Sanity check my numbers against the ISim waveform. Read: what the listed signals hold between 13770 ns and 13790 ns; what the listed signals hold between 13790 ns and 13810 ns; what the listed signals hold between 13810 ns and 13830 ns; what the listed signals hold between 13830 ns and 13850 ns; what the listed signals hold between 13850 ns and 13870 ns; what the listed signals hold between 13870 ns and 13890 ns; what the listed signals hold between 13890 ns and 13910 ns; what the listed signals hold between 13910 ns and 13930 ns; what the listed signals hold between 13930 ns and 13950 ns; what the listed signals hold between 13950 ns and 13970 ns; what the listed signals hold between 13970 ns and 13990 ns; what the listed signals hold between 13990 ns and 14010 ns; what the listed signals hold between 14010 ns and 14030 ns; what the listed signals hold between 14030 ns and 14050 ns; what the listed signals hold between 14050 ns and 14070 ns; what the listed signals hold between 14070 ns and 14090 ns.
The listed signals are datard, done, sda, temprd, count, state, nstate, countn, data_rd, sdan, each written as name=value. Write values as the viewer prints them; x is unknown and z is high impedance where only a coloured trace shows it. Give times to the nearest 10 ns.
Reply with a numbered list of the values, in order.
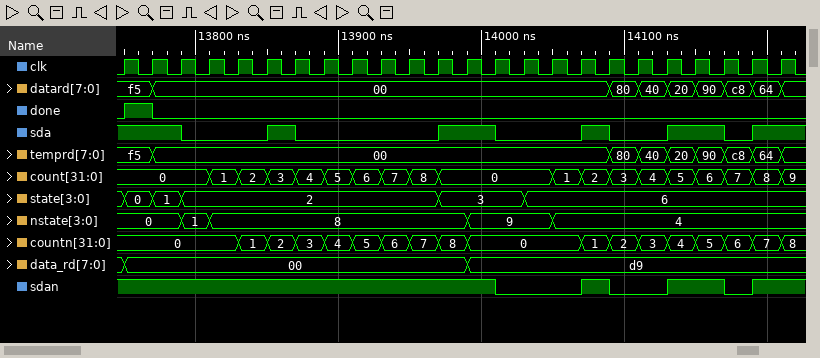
1. datard=00, done=0, sda=1, temprd=00, count=0, state=1, nstate=0, countn=0, data_rd=00, sdan=1
2. datard=00, done=0, sda=0, temprd=00, count=0, state=2, nstate=1, countn=0, data_rd=00, sdan=1
3. datard=00, done=0, sda=0, temprd=00, count=1, state=2, nstate=8, countn=0, data_rd=00, sdan=1
4. datard=00, done=0, sda=0, temprd=00, count=2, state=2, nstate=8, countn=1, data_rd=00, sdan=1
5. datard=00, done=0, sda=1, temprd=00, count=3, state=2, nstate=8, countn=2, data_rd=00, sdan=1
6. datard=00, done=0, sda=0, temprd=00, count=4, state=2, nstate=8, countn=3, data_rd=00, sdan=1
7. datard=00, done=0, sda=0, temprd=00, count=5, state=2, nstate=8, countn=4, data_rd=00, sdan=1
8. datard=00, done=0, sda=0, temprd=00, count=6, state=2, nstate=8, countn=5, data_rd=00, sdan=1
9. datard=00, done=0, sda=0, temprd=00, count=7, state=2, nstate=8, countn=6, data_rd=00, sdan=1
10. datard=00, done=0, sda=0, temprd=00, count=8, state=2, nstate=8, countn=7, data_rd=00, sdan=1
11. datard=00, done=0, sda=1, temprd=00, count=0, state=3, nstate=8, countn=8, data_rd=00, sdan=1
12. datard=00, done=0, sda=1, temprd=00, count=0, state=3, nstate=9, countn=0, data_rd=d9, sdan=1
13. datard=00, done=0, sda=0, temprd=00, count=0, state=3, nstate=9, countn=0, data_rd=d9, sdan=0
14. datard=00, done=0, sda=0, temprd=00, count=0, state=6, nstate=9, countn=0, data_rd=d9, sdan=0
15. datard=00, done=0, sda=0, temprd=00, count=1, state=6, nstate=4, countn=0, data_rd=d9, sdan=0
16. datard=00, done=0, sda=1, temprd=00, count=2, state=6, nstate=4, countn=1, data_rd=d9, sdan=1
